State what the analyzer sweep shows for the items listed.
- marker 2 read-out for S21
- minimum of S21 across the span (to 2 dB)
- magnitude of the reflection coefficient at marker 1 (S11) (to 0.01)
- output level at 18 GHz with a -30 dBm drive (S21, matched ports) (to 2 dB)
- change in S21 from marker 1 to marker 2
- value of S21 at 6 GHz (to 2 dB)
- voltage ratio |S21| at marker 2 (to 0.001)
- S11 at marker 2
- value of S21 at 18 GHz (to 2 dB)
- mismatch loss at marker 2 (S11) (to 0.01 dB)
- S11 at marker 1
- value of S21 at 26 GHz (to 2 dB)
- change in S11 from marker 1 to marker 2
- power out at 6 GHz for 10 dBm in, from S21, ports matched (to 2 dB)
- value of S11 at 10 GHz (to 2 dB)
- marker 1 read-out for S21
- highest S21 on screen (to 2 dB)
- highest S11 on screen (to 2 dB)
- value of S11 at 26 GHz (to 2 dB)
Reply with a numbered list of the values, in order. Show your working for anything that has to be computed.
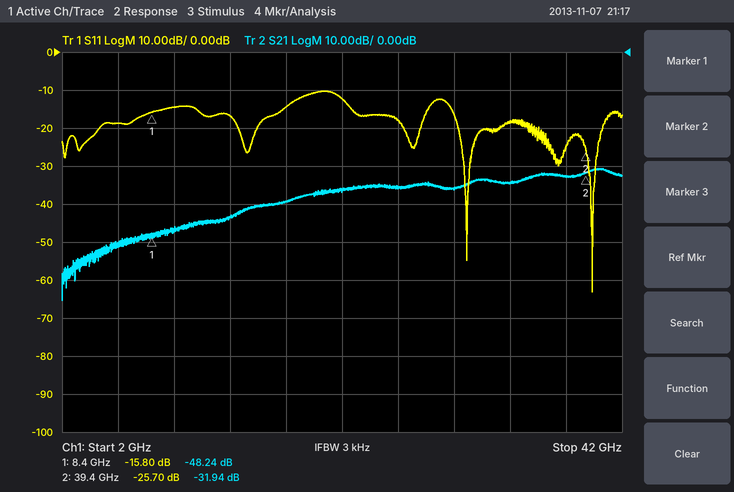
1. -31.94 dB
2. -66 dB
3. 10^(-15.8/20) ≈ 0.16
4. -30 dBm + (-40 dB) = -70 dBm
5. -31.94 − (-48.24) = 16.30 dB
6. -50 dB
7. 10^(-31.94/20) ≈ 0.025
8. -25.70 dB
9. -40 dB
10. −10 log10(1 − 10^(-25.7/10)) ≈ 0.01 dB
11. -15.80 dB
12. -36 dB
13. -25.7 − (-15.8) = -9.90 dB
14. 10 dBm + (-50 dB) = -40 dBm
15. -14 dB
16. -48.24 dB
17. -30 dB
18. -10 dB
19. -18 dB
